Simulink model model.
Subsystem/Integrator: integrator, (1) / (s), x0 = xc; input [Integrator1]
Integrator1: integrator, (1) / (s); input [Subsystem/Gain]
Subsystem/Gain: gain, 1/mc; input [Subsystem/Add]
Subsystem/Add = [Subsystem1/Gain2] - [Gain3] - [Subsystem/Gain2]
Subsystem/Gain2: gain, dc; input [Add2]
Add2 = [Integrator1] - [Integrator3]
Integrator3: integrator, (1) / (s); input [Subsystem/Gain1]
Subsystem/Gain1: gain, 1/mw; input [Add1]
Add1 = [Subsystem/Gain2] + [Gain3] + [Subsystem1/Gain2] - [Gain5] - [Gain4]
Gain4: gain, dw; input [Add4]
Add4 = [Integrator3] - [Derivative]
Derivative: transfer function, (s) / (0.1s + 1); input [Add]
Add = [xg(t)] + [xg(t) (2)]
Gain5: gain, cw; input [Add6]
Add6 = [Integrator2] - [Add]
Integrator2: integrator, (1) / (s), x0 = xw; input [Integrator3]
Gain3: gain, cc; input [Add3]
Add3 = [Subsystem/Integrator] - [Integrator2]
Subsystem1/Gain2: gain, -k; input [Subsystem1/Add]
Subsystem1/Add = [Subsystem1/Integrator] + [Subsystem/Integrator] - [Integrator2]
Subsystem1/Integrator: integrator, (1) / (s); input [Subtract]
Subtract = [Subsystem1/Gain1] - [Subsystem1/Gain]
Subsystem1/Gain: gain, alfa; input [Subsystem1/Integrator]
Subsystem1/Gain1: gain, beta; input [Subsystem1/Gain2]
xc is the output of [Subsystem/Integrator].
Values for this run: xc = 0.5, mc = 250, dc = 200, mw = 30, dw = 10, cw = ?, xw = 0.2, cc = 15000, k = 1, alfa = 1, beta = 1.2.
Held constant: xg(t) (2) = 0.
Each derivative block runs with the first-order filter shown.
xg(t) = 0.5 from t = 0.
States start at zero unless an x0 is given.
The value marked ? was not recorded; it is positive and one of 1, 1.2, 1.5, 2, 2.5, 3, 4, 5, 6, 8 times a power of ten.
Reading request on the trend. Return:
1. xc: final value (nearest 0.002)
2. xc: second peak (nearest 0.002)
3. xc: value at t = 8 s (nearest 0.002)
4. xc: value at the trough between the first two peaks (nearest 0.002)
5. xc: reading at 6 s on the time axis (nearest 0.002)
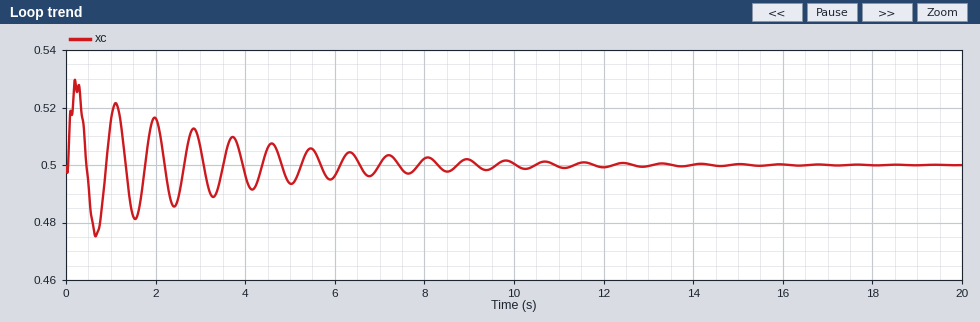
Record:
0.500
0.522
0.502
0.476
0.496
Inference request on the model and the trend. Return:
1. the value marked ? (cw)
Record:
100000
